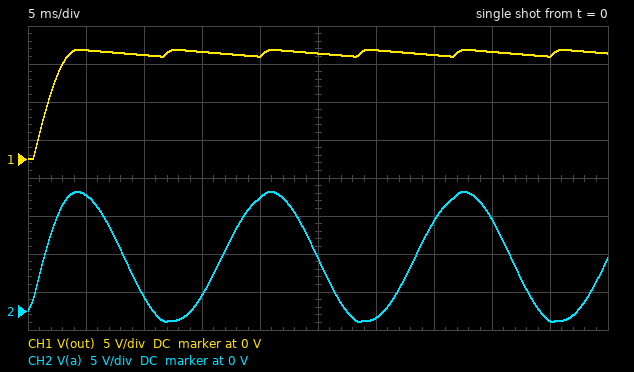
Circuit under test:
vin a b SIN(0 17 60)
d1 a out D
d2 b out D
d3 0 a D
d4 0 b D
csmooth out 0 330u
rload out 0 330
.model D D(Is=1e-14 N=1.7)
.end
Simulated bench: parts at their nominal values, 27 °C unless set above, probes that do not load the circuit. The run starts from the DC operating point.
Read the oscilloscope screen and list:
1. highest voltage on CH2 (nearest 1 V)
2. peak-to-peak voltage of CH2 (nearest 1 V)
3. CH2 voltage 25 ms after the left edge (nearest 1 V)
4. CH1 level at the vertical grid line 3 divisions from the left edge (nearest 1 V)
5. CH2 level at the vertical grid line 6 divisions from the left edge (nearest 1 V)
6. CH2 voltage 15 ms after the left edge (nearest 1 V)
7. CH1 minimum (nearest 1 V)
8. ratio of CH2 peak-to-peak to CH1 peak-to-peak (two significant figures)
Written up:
16 V
17 V
7 V
14 V
-1 V
2 V
0 V
1.2
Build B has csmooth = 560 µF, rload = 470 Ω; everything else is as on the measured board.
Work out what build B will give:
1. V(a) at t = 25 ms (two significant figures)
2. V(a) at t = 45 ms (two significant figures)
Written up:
7.1 V
-1.1 V
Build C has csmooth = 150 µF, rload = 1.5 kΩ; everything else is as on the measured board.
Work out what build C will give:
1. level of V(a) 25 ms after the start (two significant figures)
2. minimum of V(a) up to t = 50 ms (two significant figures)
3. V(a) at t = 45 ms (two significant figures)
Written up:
7.1 V
-1.3 V
-1.1 V
